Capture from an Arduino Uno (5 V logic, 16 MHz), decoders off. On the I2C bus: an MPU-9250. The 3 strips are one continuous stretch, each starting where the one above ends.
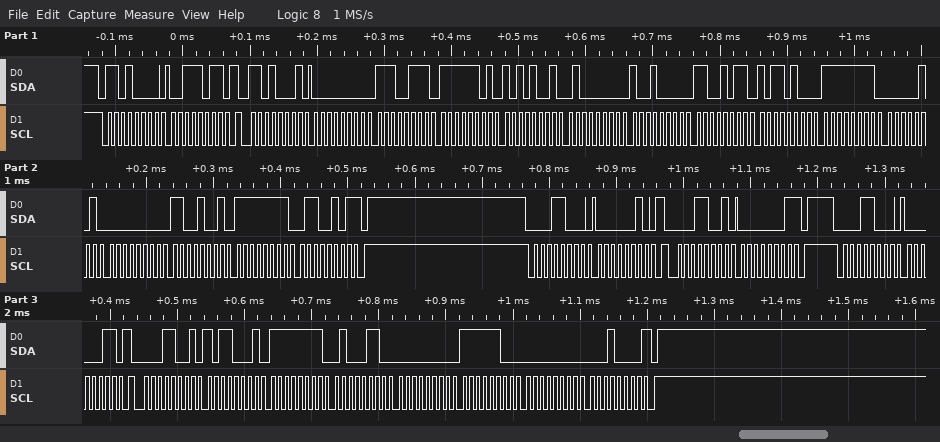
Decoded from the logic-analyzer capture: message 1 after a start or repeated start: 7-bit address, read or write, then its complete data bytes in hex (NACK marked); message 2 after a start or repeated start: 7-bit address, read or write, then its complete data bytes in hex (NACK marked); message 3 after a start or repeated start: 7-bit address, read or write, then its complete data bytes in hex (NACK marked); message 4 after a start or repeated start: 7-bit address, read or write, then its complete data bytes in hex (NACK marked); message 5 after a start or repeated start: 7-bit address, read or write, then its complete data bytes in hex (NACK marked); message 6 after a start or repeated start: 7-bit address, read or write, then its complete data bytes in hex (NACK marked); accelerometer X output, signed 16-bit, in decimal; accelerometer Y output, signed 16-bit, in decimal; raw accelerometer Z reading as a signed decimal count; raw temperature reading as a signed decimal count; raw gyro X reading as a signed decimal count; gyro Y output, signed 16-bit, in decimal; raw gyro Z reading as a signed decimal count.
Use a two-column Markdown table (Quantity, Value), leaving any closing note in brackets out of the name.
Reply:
| Quantity | Value |
|---|---|
| message 1 after a start or repeated start: 7-bit address, read or write, then its complete data bytes in hex | 0x68 write: 3B |
| message 2 after a start or repeated start: 7-bit address, read or write, then its complete data bytes in hex | 0x68 read: 00 E7 FD A9 40 90 CB B4 FF 05 00 C9 FF 65 NACK |
| message 3 after a start or repeated start: 7-bit address, read or write, then its complete data bytes in hex | 0x0C write: 02 |
| message 4 after a start or repeated start: 7-bit address, read or write, then its complete data bytes in hex | 0x0C read: 01 NACK |
| message 5 after a start or repeated start: 7-bit address, read or write, then its complete data bytes in hex | 0x0C write: 03 |
| message 6 after a start or repeated start: 7-bit address, read or write, then its complete data bytes in hex | 0x0C read: B1 FF 46 00 FC 00 10 NACK |
| accelerometer X output, signed 16-bit, in decimal | 231 |
| accelerometer Y output, signed 16-bit, in decimal | -599 |
| raw accelerometer Z reading as a signed decimal count | 16528 |
| raw temperature reading as a signed decimal count | -13388 |
| raw gyro X reading as a signed decimal count | -251 |
| gyro Y output, signed 16-bit, in decimal | 201 |
| raw gyro Z reading as a signed decimal count | -155 |
